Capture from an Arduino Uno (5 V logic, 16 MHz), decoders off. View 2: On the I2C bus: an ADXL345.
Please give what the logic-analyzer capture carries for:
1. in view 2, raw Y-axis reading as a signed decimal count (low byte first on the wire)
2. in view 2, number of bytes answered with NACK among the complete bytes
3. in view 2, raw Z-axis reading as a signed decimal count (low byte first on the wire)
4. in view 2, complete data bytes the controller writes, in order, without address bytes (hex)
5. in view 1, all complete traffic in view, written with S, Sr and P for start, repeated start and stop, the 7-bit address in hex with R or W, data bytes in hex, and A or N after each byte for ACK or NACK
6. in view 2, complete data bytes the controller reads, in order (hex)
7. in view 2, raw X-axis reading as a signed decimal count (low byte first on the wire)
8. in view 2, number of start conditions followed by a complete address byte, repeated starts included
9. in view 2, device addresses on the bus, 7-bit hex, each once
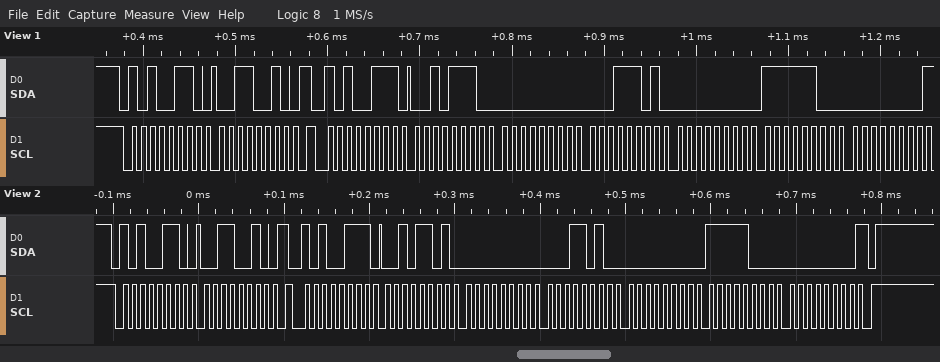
26
1
248
32
S 53W A 32 A Sr 53R A 2E A 00 A 1D A 00 A FC A 00 N
2D 00 1A 00 F8 00
45
2
0x53
